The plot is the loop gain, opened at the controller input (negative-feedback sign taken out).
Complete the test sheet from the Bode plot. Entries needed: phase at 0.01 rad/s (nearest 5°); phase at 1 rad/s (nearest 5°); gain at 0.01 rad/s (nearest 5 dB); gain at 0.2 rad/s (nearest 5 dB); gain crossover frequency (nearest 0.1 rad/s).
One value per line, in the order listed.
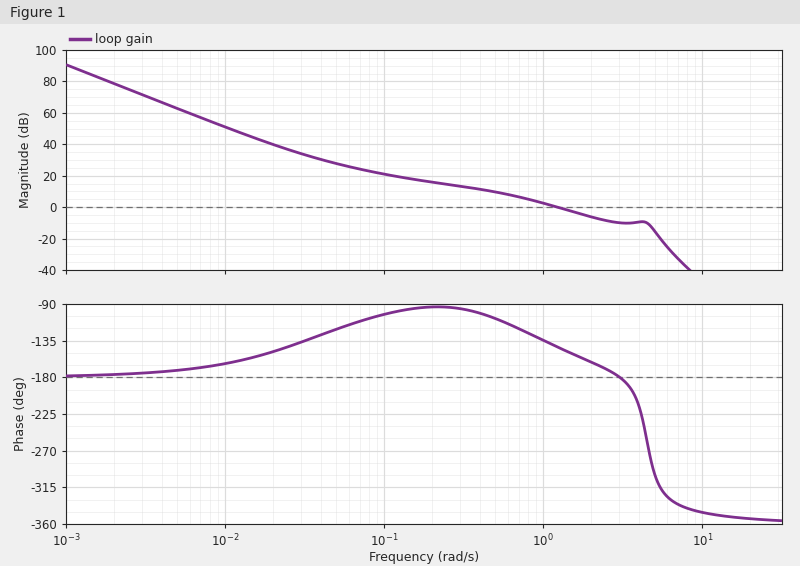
-165°
-135°
50 dB
15 dB
1.2 rad/s
